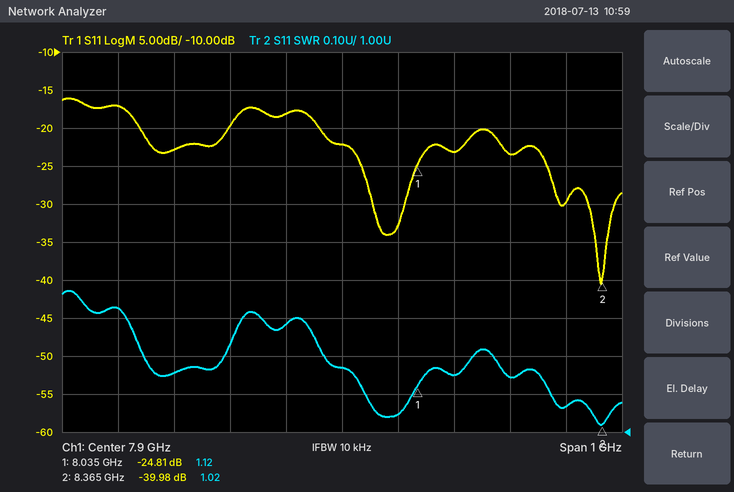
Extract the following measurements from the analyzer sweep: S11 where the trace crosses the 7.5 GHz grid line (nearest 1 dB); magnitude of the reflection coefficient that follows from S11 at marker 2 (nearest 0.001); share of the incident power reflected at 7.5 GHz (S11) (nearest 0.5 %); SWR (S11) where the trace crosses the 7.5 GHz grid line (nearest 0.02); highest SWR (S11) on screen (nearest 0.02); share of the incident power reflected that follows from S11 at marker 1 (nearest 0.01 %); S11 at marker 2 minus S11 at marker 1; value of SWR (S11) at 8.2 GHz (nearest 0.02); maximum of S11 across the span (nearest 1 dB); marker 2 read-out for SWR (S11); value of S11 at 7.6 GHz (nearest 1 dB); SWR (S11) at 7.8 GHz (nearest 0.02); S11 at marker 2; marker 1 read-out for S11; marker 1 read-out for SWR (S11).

-17 dB
0.010
2.0 %
1.32
1.38
0.33 %
-15.17 dB
1.14
-16 dB
1.02
-23 dB
1.28
-39.98 dB
-24.81 dB
1.12
